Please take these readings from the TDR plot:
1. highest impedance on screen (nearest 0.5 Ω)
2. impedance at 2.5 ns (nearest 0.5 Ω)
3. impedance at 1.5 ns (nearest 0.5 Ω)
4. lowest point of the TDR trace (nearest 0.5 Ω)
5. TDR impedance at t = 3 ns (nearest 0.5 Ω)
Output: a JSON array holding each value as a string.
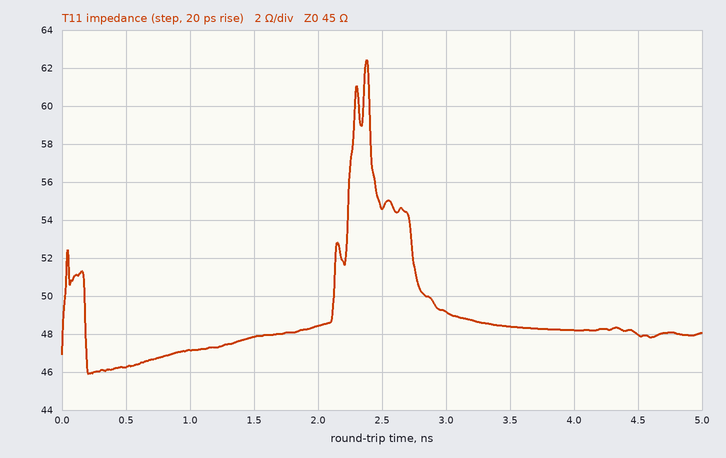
["62.5 Ω", "54.5 Ω", "48.0 Ω", "46.0 Ω", "49.0 Ω"]
